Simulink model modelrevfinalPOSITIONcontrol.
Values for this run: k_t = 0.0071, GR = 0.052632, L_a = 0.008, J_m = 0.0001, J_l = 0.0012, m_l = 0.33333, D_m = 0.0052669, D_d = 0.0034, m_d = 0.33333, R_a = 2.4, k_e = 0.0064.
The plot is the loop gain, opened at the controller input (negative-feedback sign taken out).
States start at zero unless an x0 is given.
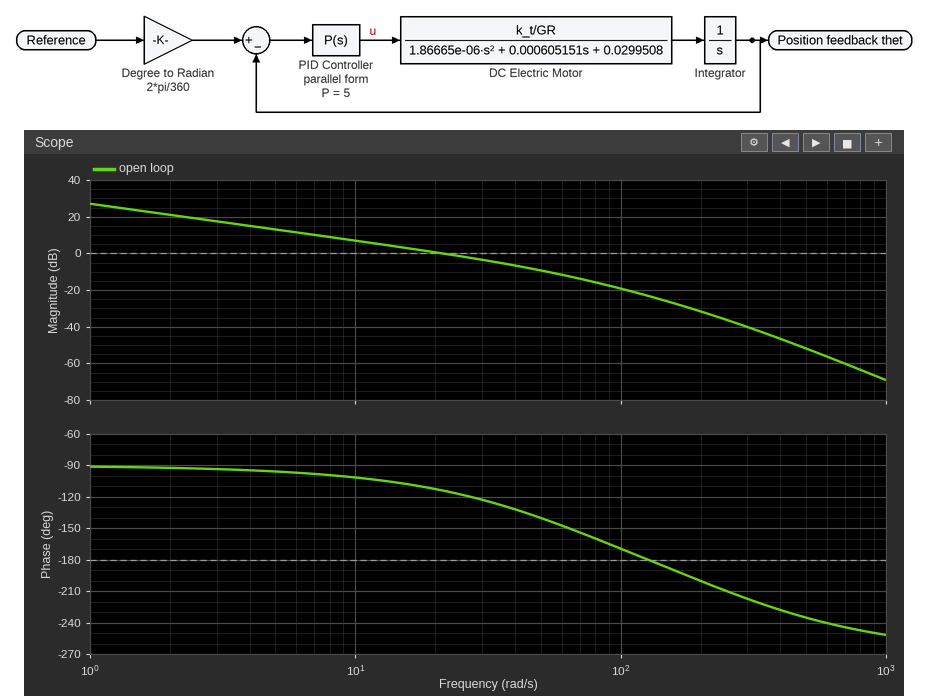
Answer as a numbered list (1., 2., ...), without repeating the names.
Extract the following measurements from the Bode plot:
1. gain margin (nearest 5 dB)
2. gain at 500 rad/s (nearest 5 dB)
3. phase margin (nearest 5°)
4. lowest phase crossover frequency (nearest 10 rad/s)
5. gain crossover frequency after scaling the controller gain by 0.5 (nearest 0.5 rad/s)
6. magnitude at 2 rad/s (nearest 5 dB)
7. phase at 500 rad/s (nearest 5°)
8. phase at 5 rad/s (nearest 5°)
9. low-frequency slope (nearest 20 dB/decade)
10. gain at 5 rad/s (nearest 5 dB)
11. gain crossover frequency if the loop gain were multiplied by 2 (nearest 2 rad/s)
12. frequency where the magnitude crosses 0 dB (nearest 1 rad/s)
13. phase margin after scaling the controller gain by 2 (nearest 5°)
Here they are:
1. 25 dB
2. -50 dB
3. 65°
4. 130 rad/s
5. 11.0 rad/s
6. 20 dB
7. -235°
8. -95°
9. -20 dB/decade
10. 15 dB
11. 38 rad/s
12. 21 rad/s
13. 50°
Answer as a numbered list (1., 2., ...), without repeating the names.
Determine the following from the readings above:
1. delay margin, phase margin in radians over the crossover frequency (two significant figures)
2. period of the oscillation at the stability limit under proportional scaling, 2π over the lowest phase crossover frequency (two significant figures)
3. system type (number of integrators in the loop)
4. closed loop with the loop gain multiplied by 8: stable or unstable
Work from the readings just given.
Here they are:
1. 0.054 s
2. 0.048 s
3. 1
4. stable
